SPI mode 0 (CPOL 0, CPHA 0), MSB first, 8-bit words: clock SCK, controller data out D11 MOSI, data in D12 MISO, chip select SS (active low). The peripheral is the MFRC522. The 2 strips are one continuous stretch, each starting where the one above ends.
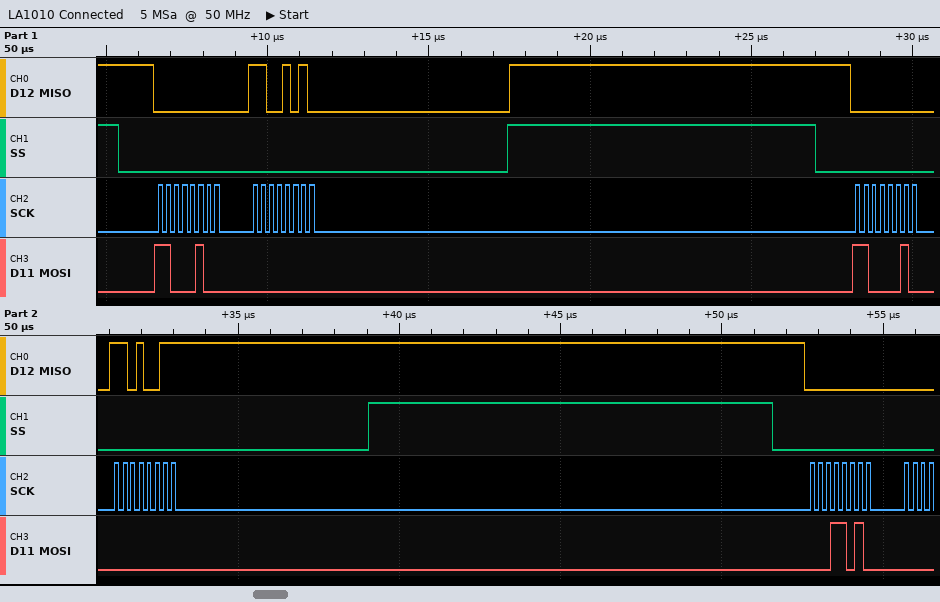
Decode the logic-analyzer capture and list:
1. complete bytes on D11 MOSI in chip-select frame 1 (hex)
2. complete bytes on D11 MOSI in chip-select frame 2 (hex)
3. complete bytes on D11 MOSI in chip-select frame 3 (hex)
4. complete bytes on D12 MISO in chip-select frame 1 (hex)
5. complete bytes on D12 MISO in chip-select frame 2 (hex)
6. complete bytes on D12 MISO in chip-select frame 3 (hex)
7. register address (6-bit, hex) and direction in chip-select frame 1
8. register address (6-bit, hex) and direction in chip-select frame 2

C4 00
C2 00
1A
00 CA
00 D3
00
0x22 read
0x21 read
